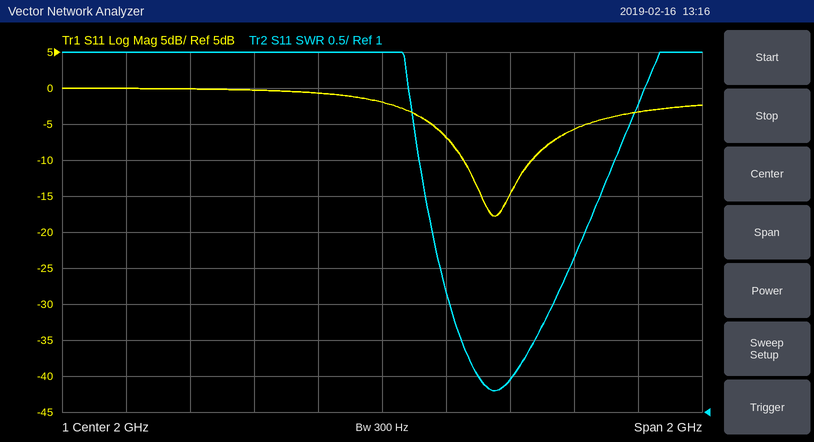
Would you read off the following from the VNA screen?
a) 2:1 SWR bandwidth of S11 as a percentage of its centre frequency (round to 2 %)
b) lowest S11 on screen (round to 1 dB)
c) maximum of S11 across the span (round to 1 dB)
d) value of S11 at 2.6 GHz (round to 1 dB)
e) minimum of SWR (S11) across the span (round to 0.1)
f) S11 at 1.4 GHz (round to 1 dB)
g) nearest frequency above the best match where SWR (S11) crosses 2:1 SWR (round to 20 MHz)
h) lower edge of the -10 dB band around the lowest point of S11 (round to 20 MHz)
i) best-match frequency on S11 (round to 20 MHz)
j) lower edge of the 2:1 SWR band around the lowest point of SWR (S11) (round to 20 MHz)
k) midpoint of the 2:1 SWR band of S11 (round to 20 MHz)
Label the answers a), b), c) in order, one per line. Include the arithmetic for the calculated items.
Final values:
a) 240 MHz / 2.36 GHz ≈ 10 %
b) -18 dB
c) 0 dB
d) -6 dB
e) 1.3
f) 0 dB
g) 2.48 GHz
h) 2.26 GHz
i) 2.36 GHz
j) 2.24 GHz
k) 2.36 GHz
